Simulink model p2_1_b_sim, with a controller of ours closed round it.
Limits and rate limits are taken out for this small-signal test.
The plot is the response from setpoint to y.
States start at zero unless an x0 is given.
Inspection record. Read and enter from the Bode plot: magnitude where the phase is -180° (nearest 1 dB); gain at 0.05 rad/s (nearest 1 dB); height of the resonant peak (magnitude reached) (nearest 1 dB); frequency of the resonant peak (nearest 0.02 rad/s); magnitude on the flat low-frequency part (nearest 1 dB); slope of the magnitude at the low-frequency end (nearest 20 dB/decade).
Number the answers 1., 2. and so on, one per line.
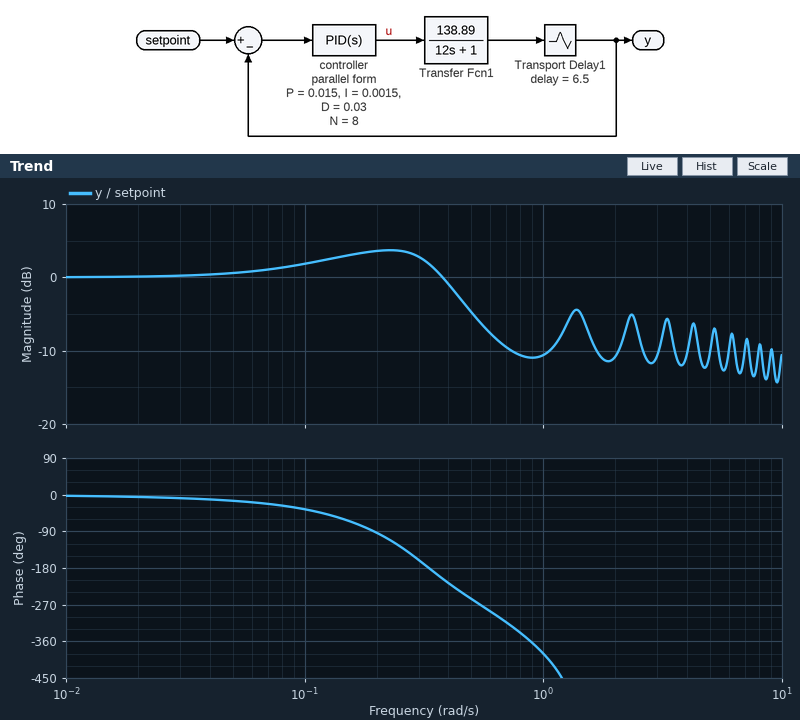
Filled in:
1. 2 dB
2. 1 dB
3. 4 dB
4. 0.22 rad/s
5. 0 dB
6. 0 dB/decade
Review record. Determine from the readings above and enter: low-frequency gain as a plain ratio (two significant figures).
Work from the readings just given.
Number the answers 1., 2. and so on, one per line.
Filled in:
1. 1.0
